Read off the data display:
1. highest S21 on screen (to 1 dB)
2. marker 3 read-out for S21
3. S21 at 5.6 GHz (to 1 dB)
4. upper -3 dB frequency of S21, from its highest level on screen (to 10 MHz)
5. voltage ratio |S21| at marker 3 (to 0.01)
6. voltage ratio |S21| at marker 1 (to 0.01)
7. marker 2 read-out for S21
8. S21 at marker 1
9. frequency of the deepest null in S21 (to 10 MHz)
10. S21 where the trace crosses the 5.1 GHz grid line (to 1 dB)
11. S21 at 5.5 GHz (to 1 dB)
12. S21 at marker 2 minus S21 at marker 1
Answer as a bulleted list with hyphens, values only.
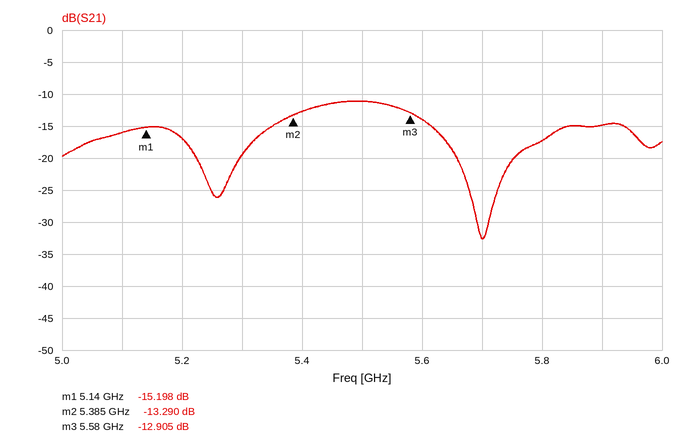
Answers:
- -11 dB
- -12.905 dB
- -14 dB
- 5.60 GHz
- 0.23
- 0.17
- -13.290 dB
- -15.198 dB
- 5.70 GHz
- -16 dB
- -11 dB
- 1.908 dB
